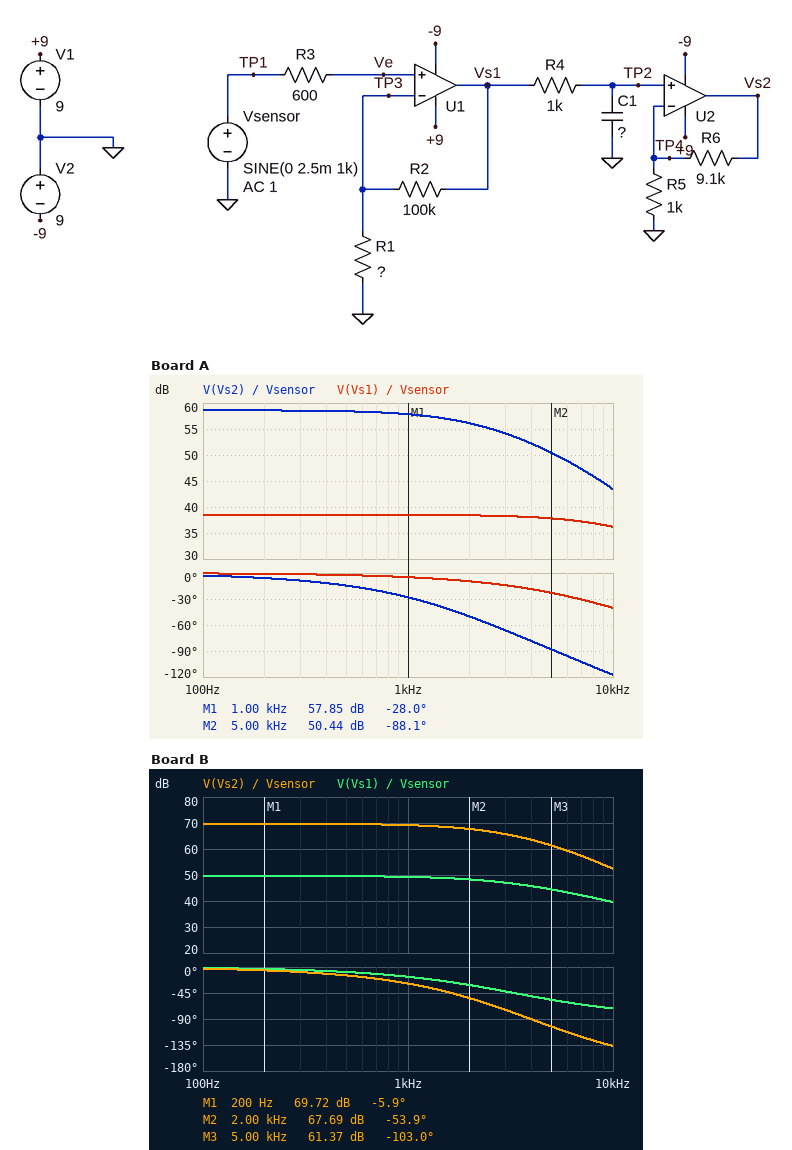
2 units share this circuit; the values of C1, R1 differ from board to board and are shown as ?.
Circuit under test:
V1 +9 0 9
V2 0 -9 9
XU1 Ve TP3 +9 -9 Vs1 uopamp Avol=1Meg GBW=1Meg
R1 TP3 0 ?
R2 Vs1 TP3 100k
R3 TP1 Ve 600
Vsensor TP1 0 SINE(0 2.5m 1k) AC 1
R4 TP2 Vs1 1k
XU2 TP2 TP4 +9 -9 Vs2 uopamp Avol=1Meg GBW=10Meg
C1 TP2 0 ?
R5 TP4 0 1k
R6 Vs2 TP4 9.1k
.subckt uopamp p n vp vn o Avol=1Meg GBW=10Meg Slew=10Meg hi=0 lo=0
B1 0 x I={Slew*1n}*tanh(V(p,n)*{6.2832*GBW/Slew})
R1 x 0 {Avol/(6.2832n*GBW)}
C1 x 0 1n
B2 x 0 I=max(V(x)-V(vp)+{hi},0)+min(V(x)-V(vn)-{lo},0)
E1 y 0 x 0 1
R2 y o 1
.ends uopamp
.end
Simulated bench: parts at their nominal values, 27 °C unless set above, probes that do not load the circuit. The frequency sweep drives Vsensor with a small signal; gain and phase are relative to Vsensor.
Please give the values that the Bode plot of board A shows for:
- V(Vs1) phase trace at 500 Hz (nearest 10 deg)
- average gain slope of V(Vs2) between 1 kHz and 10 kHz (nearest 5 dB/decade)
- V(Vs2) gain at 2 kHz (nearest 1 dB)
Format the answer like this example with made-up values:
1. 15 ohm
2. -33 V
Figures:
1. 0 deg
2. -15 dB/decade
3. 56 dB
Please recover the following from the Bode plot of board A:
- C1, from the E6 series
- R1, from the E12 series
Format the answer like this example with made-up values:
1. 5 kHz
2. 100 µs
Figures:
1. 68 nF
2. 1.2 kΩ
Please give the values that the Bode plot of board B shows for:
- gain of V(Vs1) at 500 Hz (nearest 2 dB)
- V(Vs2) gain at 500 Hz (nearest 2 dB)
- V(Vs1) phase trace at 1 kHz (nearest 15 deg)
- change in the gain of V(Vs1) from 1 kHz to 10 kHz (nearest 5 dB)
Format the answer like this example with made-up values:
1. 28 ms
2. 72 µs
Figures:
1. 50 dB
2. 70 dB
3. -15 deg
4. -10 dB
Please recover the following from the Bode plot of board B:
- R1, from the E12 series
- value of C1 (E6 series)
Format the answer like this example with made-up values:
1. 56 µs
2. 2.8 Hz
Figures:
1. 330 Ω
2. 33 nF
